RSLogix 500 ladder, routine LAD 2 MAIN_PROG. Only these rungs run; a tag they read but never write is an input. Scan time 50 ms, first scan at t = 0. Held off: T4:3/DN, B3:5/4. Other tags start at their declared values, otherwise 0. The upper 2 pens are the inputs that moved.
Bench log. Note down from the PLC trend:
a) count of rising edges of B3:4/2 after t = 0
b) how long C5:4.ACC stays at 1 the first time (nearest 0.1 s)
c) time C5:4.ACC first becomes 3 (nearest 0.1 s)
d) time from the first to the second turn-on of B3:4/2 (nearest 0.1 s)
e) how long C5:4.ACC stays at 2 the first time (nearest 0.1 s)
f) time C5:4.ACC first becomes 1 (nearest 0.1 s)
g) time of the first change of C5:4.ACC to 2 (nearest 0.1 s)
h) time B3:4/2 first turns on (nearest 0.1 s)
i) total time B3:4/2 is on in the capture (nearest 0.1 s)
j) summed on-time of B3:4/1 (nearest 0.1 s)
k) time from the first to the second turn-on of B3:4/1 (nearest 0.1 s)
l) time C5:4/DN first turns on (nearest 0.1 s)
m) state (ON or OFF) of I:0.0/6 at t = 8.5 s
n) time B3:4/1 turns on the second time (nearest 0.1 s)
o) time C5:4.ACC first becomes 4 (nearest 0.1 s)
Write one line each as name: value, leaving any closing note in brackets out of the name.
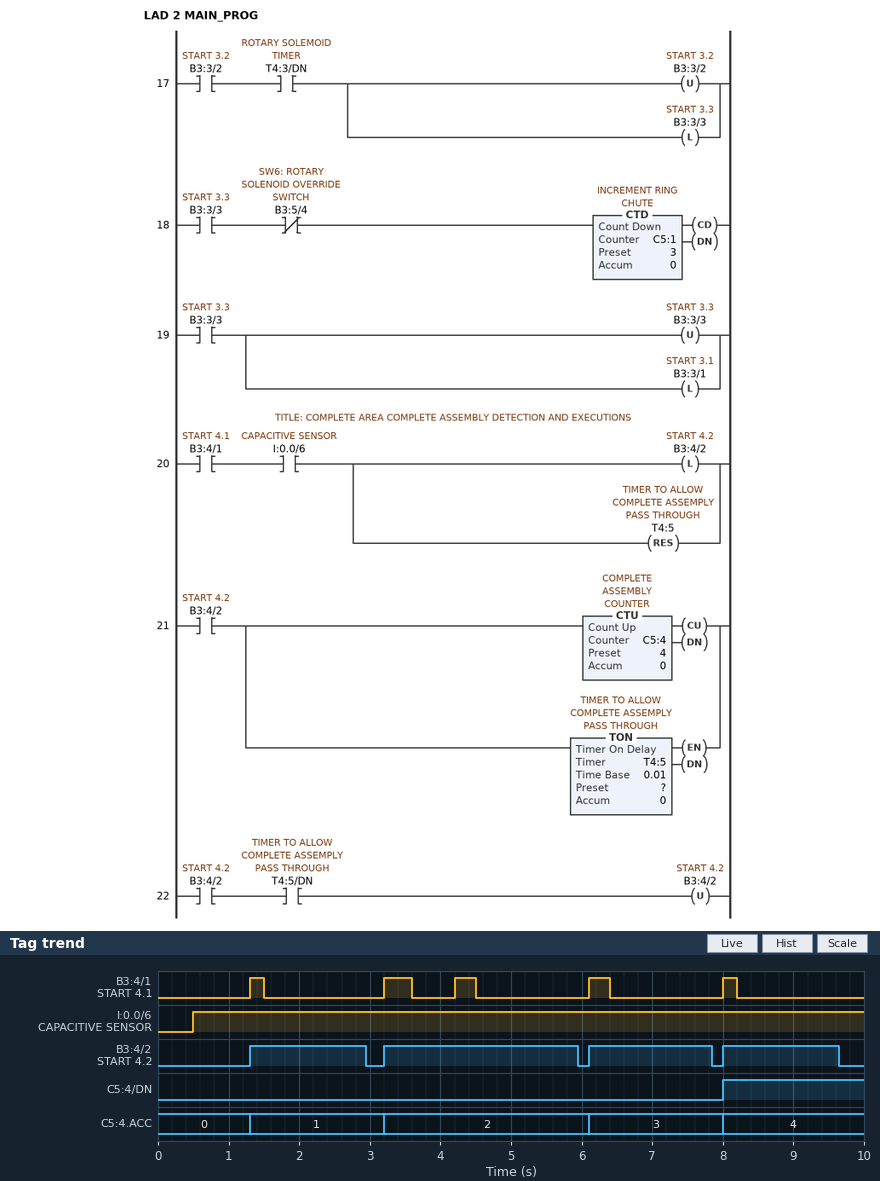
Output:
count of rising edges of B3:4/2 after t = 0: 4
how long C5:4.ACC stays at 1 the first time: 1.9 s
time C5:4.ACC first becomes 3: 6.1 s
time from the first to the second turn-on of B3:4/2: 1.9 s
how long C5:4.ACC stays at 2 the first time: 2.9 s
time C5:4.ACC first becomes 1: 1.3 s
time of the first change of C5:4.ACC to 2: 3.2 s
time B3:4/2 first turns on: 1.3 s
total time B3:4/2 is on in the capture: 7.8 s
summed on-time of B3:4/1: 1.4 s
time from the first to the second turn-on of B3:4/1: 1.9 s
time C5:4/DN first turns on: 8.0 s
state (ON or OFF) of I:0.0/6 at t = 8.5 s: ON
time B3:4/1 turns on the second time: 3.2 s
time C5:4.ACC first becomes 4: 8.0 s
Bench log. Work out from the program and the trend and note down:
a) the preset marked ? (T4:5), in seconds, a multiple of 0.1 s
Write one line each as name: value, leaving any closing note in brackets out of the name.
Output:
the preset marked ? (T4:5), in seconds, a multiple of 0.1 s: 1.5 s
